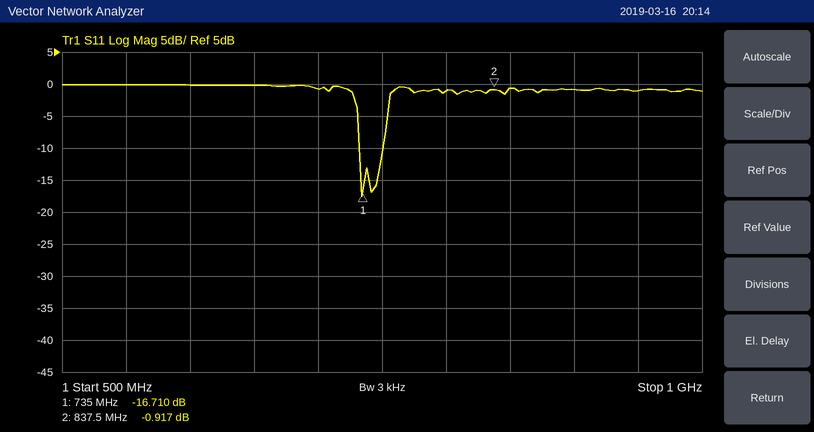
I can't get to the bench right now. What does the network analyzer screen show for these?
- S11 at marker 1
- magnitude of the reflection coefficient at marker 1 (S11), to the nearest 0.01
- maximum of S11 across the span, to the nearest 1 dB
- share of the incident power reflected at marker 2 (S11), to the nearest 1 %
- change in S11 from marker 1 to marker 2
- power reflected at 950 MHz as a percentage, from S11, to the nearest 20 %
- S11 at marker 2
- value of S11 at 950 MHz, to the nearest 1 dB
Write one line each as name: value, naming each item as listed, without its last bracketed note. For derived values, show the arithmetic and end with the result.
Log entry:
S11 at marker 1: -16.710 dB
magnitude of the reflection coefficient at marker 1 (S11), to the nearest 0.01: 10^(-16.71/20) ≈ 0.15
maximum of S11 across the span, to the nearest 1 dB: 0 dB
share of the incident power reflected at marker 2 (S11), to the nearest 1 %: 10^(-0.917/10) ≈ 81 %
change in S11 from marker 1 to marker 2: -0.917 − (-16.71) = 15.793 dB
power reflected at 950 MHz as a percentage, from S11, to the nearest 20 %: 10^(-1/10) ≈ 79.4 %, so 80 % to the nearest 20 %
S11 at marker 2: -0.917 dB
value of S11 at 950 MHz, to the nearest 1 dB: -1 dB
